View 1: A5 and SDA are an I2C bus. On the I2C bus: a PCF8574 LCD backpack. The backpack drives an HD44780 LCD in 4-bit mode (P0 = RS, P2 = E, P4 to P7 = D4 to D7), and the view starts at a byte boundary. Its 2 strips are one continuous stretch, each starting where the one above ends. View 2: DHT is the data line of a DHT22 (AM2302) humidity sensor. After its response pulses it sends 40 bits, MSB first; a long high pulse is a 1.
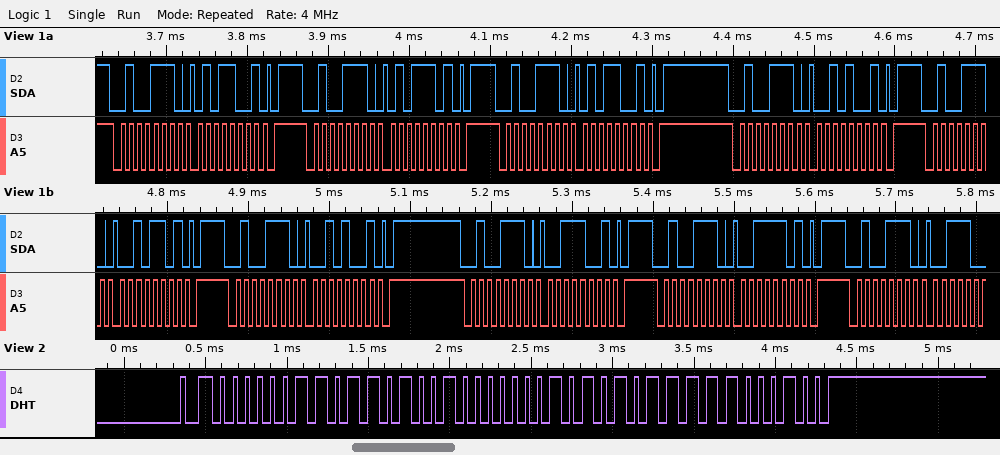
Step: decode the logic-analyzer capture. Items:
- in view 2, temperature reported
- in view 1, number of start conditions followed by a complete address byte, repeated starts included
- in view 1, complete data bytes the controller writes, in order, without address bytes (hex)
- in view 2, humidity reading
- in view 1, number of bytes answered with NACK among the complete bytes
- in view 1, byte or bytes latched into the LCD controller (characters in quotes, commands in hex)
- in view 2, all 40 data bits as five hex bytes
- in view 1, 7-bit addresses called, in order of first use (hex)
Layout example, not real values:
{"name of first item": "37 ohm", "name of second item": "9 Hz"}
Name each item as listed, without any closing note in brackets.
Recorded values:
{"in view 2, temperature reported": "34.3 °C", "in view 1, number of start conditions followed by a complete address byte, repeated starts included": "9", "in view 1, complete data bytes the controller writes, in order, without address bytes": "59 5D 59 29 2D 29 39 3D", "in view 2, humidity reading": "87.3 %", "in view 1, number of bytes answered with NACK among the complete bytes": "0", "in view 1, byte or bytes latched into the LCD controller": "'R'", "in view 2, all 40 data bits as five hex bytes": "03 69 01 57 C4", "in view 1, 7-bit addresses called, in order of first use": "0x27"}
